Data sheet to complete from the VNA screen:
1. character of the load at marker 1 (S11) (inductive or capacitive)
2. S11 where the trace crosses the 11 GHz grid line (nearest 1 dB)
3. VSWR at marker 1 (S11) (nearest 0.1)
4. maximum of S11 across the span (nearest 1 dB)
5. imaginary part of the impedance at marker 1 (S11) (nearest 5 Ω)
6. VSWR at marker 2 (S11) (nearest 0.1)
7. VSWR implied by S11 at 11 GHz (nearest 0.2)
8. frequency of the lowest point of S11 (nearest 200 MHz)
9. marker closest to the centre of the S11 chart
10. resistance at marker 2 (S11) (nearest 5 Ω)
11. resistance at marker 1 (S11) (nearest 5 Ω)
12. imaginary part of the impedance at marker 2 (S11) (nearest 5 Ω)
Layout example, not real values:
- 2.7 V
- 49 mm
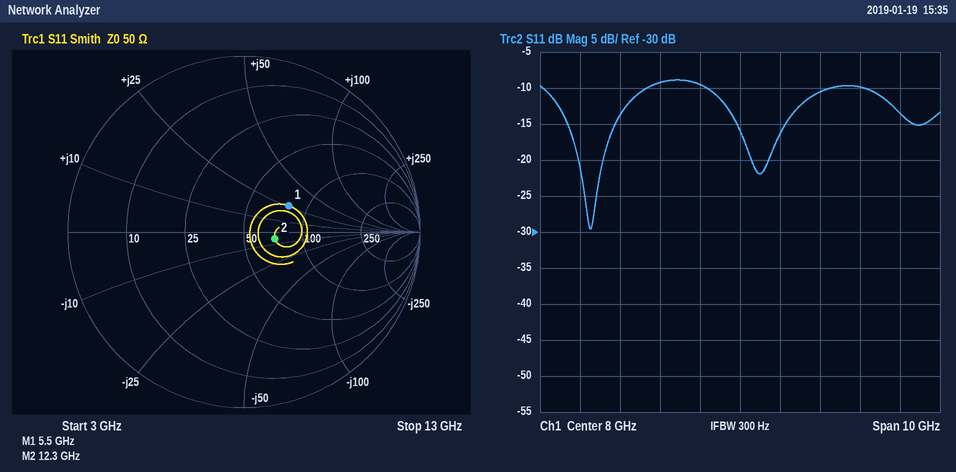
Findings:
- inductive
- -10 dB
- 1.8
- -9 dB
- +25 Ω
- 1.4
- 2.0
- 4.2 GHz
- marker 2
- 70 Ω
- 80 Ω
- -5 Ω
